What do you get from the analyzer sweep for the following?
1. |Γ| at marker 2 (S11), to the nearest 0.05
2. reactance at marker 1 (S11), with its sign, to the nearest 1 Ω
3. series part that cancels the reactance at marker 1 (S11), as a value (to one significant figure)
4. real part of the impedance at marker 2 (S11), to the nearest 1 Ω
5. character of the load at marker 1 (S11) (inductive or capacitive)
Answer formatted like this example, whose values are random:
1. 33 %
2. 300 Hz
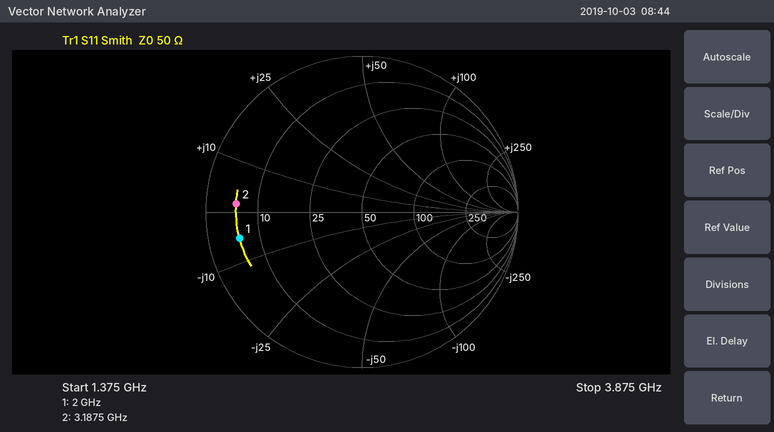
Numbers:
1. 0.80
2. -5 Ω
3. 400 pH
4. 5 Ω
5. capacitive
